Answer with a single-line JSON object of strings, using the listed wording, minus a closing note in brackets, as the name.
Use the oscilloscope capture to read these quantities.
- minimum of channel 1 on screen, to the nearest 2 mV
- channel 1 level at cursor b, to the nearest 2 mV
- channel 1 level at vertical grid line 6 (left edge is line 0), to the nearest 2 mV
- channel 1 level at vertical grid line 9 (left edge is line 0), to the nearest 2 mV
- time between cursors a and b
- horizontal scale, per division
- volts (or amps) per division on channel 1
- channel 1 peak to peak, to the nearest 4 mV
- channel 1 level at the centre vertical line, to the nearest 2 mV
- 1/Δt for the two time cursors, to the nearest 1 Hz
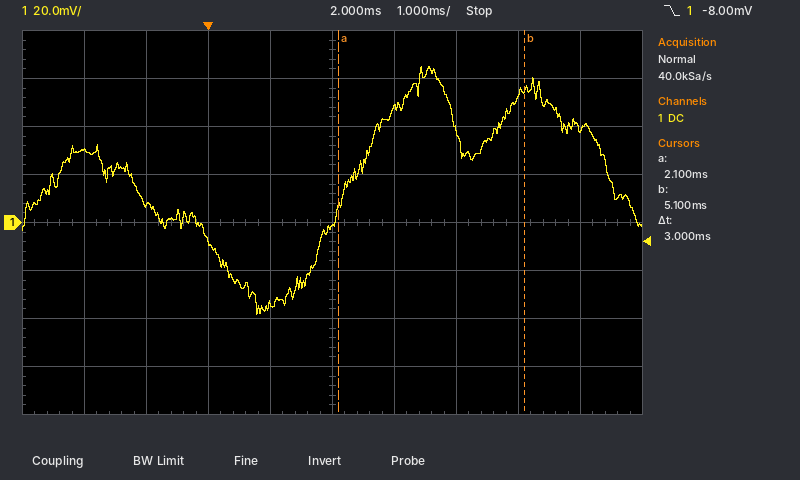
{"minimum of channel 1 on screen, to the nearest 2 mV": "-38 mV", "channel 1 level at cursor b, to the nearest 2 mV": "56 mV", "channel 1 level at vertical grid line 6 (left edge is line 0), to the nearest 2 mV": "48 mV", "channel 1 level at vertical grid line 9 (left edge is line 0), to the nearest 2 mV": "40 mV", "time between cursors a and b": "3 ms", "horizontal scale, per division": "1 ms", "volts (or amps) per division on channel 1": "20 mV", "channel 1 peak to peak, to the nearest 4 mV": "104 mV", "channel 1 level at the centre vertical line, to the nearest 2 mV": "-2 mV", "1/Δt for the two time cursors, to the nearest 1 Hz": "333 Hz"}
